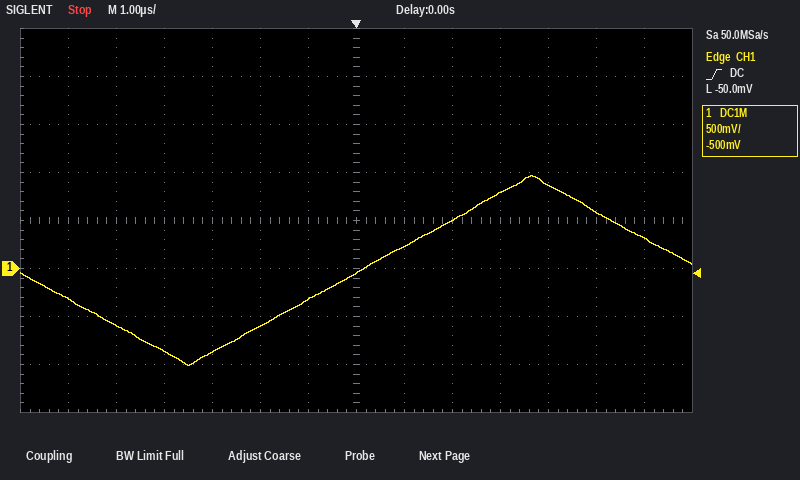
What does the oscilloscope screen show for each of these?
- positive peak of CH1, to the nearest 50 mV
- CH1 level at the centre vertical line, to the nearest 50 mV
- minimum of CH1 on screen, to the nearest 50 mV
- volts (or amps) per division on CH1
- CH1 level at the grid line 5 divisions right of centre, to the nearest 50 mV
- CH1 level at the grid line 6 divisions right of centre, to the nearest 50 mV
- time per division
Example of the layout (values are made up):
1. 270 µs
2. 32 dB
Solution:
1. 950 mV
2. -50 mV
3. -1.00 V
4. 500 mV
5. 600 mV
6. 300 mV
7. 1 µs
